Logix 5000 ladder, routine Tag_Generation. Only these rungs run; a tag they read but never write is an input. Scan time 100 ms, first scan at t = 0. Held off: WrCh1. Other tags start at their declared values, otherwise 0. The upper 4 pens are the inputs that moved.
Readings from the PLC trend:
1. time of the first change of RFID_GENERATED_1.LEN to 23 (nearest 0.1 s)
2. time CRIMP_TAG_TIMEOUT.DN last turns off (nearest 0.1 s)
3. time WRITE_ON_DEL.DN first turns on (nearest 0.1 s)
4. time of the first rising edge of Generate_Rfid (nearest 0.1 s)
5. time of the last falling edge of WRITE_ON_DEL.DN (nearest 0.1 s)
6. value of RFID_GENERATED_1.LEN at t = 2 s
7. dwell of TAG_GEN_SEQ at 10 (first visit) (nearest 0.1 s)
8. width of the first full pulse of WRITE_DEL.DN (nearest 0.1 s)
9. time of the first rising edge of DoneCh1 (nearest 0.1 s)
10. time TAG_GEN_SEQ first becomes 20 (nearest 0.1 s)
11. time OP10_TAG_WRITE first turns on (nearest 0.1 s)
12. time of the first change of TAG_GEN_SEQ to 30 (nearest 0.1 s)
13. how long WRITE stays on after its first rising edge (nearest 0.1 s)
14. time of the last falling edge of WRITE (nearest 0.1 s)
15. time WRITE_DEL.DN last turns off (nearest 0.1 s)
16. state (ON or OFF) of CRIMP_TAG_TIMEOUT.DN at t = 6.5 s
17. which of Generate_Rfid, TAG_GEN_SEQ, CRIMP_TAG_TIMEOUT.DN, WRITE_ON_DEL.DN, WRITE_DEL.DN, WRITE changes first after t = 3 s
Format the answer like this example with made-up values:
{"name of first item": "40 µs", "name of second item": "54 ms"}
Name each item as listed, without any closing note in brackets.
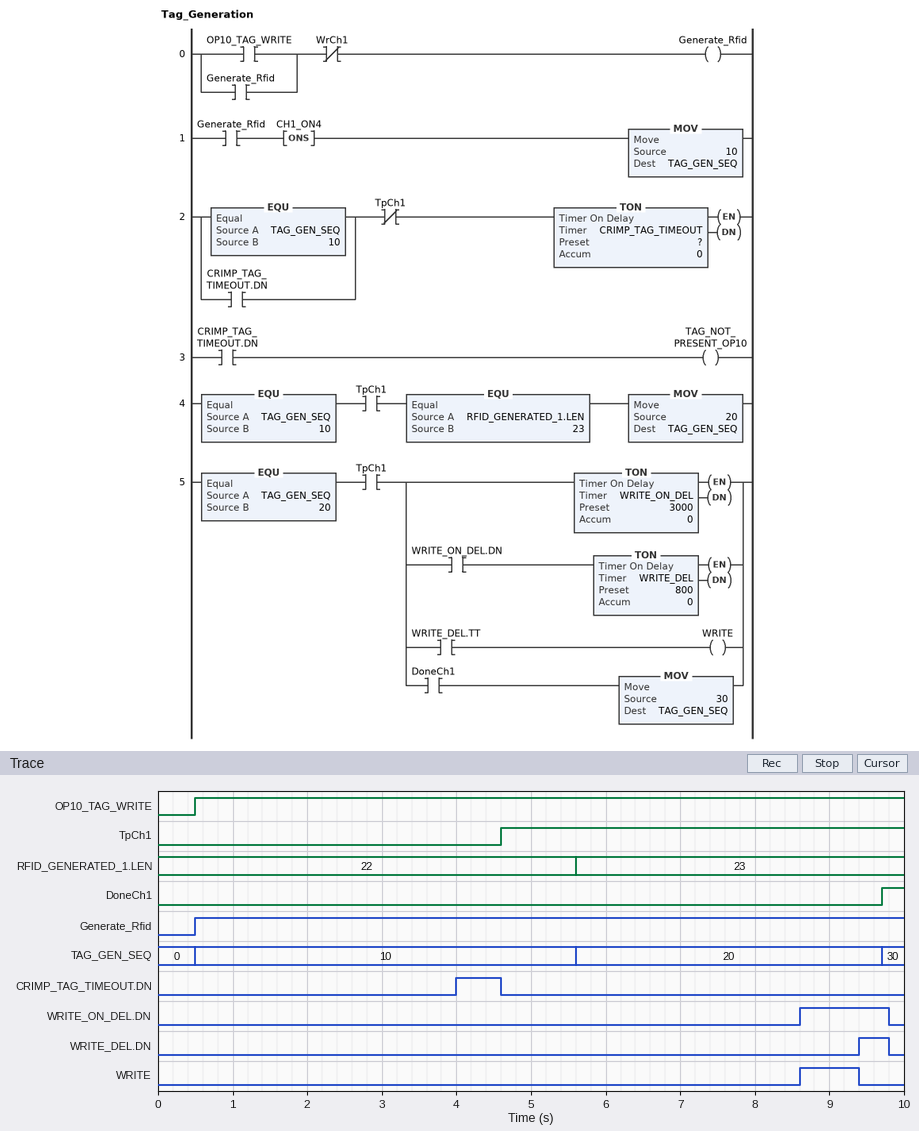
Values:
{"time of the first change of RFID_GENERATED_1.LEN to 23": "5.6 s", "time CRIMP_TAG_TIMEOUT.DN last turns off": "4.6 s", "time WRITE_ON_DEL.DN first turns on": "8.6 s", "time of the first rising edge of Generate_Rfid": "0.5 s", "time of the last falling edge of WRITE_ON_DEL.DN": "9.8 s", "value of RFID_GENERATED_1.LEN at t = 2 s": "22", "dwell of TAG_GEN_SEQ at 10 (first visit)": "5.1 s", "width of the first full pulse of WRITE_DEL.DN": "0.4 s", "time of the first rising edge of DoneCh1": "9.7 s", "time TAG_GEN_SEQ first becomes 20": "5.6 s", "time OP10_TAG_WRITE first turns on": "0.5 s", "time of the first change of TAG_GEN_SEQ to 30": "9.7 s", "how long WRITE stays on after its first rising edge": "0.8 s", "time of the last falling edge of WRITE": "9.4 s", "time WRITE_DEL.DN last turns off": "9.8 s", "state (ON or OFF) of CRIMP_TAG_TIMEOUT.DN at t = 6.5 s": "OFF", "which of Generate_Rfid, TAG_GEN_SEQ, CRIMP_TAG_TIMEOUT.DN, WRITE_ON_DEL.DN, WRITE_DEL.DN, WRITE changes first after t = 3 s": "CRIMP_TAG_TIMEOUT.DN"}
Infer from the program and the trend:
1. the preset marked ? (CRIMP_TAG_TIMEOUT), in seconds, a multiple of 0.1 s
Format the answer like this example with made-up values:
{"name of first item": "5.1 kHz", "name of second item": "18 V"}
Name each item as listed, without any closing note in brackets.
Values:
{"the preset marked ? (CRIMP_TAG_TIMEOUT), in seconds, a multiple of 0.1 s": "3.5 s"}
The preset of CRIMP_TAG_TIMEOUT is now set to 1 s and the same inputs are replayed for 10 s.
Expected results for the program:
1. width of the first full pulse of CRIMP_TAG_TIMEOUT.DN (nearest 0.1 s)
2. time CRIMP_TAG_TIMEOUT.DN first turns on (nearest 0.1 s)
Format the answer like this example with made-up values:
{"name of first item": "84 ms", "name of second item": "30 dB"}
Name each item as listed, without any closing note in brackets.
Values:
{"width of the first full pulse of CRIMP_TAG_TIMEOUT.DN": "3.1 s", "time CRIMP_TAG_TIMEOUT.DN first turns on": "1.5 s"}
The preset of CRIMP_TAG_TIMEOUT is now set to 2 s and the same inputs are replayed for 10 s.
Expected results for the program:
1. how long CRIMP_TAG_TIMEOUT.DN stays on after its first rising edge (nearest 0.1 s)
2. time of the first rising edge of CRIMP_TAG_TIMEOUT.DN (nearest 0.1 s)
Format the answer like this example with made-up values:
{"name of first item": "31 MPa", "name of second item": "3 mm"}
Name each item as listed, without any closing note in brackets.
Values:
{"how long CRIMP_TAG_TIMEOUT.DN stays on after its first rising edge": "2.1 s", "time of the first rising edge of CRIMP_TAG_TIMEOUT.DN": "2.5 s"}
